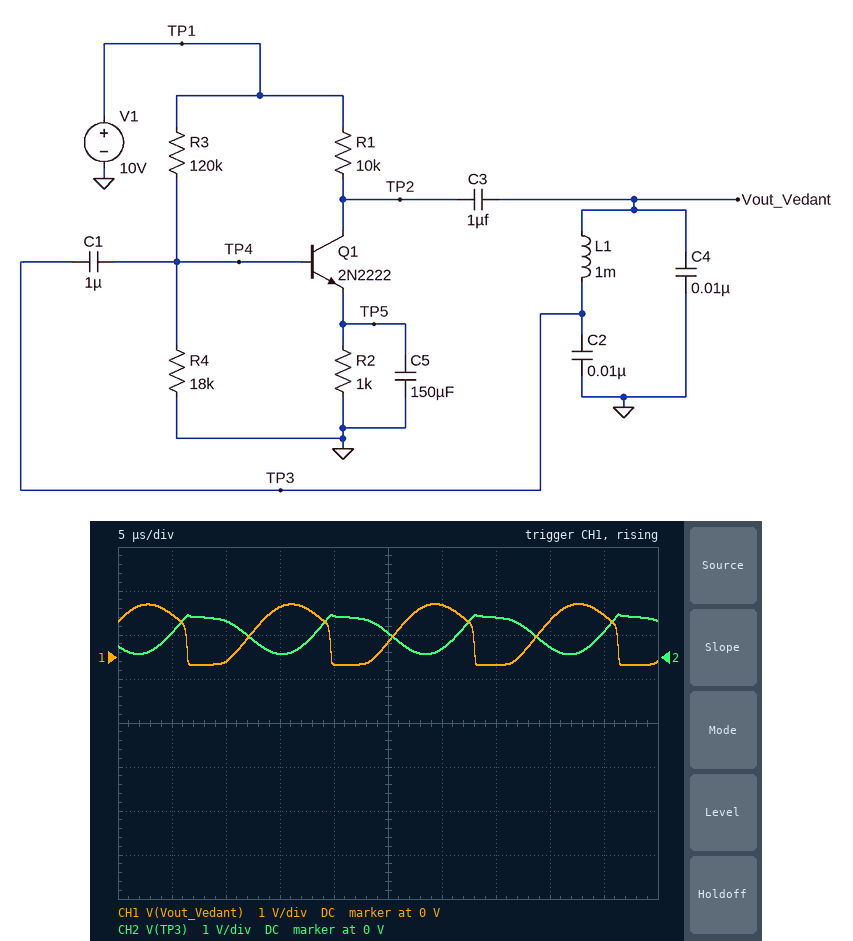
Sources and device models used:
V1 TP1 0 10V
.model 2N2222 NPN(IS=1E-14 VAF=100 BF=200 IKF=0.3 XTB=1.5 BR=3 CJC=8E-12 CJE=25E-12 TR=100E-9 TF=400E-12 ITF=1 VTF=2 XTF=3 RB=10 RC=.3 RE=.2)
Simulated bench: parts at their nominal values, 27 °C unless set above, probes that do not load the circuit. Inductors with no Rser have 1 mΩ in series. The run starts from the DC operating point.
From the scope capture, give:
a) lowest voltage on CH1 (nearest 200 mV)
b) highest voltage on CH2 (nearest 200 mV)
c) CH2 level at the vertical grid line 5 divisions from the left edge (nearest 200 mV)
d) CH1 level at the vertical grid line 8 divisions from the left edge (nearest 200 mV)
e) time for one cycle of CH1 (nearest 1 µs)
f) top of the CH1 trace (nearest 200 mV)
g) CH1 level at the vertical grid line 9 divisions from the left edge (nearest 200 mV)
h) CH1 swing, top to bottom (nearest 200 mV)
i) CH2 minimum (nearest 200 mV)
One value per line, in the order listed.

-200 mV
1.0 V
600 mV
800 mV
13 µs
1.2 V
1.0 V
1.4 V
0 V
